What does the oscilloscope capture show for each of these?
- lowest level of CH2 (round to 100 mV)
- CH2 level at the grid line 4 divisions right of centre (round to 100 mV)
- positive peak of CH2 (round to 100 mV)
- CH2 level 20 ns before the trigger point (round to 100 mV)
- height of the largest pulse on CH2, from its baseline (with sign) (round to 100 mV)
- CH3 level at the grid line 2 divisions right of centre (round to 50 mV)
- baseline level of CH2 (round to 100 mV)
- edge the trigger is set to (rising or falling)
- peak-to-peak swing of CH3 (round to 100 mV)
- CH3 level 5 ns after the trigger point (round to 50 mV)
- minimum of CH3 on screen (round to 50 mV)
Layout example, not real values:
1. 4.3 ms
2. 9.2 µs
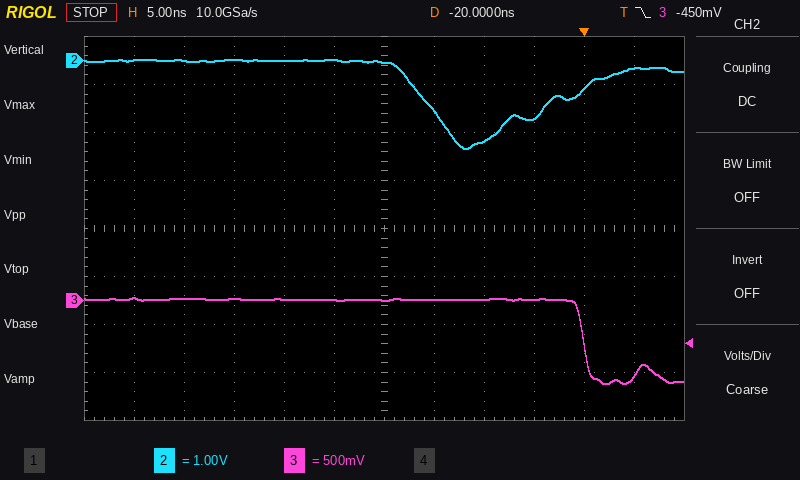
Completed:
1. -1.8 V
2. -600 mV
3. 0.0 V
4. 0.0 V
5. -1.8 V
6. 0 mV
7. 0.0 V
8. falling
9. 900 mV
10. -800 mV
11. -850 mV
